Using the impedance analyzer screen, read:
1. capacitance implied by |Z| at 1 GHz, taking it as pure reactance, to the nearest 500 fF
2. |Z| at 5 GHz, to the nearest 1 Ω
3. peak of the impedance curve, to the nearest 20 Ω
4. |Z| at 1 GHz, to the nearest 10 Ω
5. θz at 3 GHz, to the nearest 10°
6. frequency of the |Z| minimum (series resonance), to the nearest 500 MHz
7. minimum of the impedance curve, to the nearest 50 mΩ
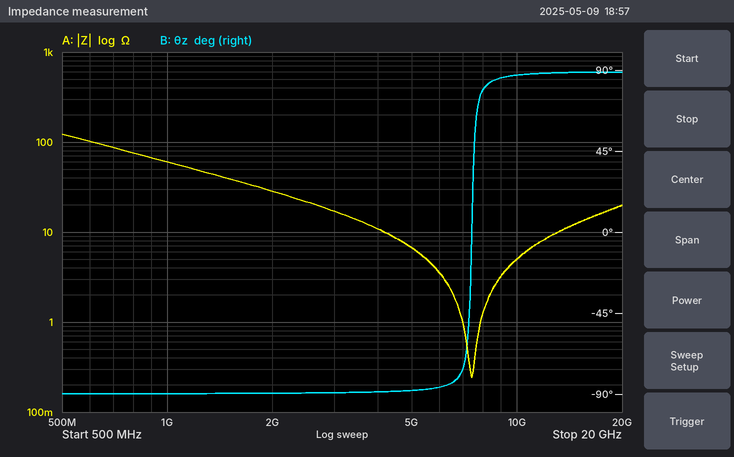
2.5 pF
7 Ω
120 Ω
60 Ω
-90°
7.5 GHz
250 mΩ
